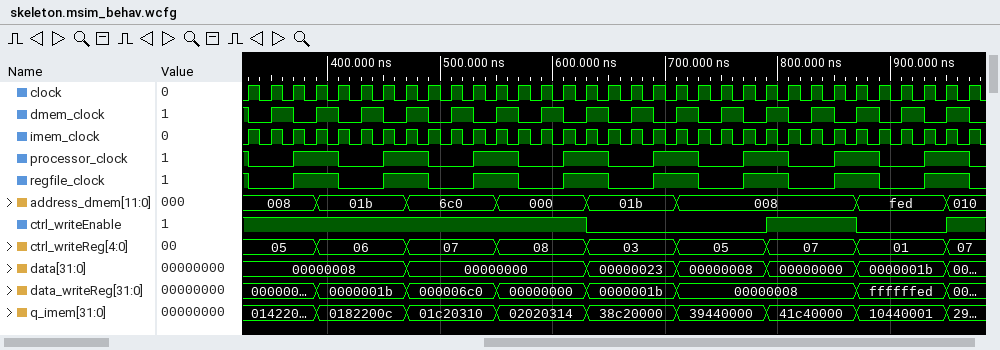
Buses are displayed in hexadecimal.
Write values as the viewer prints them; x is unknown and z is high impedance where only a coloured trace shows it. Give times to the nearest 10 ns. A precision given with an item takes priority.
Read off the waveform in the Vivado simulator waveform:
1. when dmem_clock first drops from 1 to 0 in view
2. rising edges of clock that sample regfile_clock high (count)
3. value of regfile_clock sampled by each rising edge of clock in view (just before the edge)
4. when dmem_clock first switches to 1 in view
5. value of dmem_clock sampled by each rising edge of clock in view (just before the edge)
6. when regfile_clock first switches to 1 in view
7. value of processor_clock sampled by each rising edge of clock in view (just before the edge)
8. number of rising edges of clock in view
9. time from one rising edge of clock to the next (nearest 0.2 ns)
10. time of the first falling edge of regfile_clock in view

330 ns
17
1 0 0 1 1 0 0 1 1 0 0 1 1 0 0 1 1 0 0 1 1 0 0 1 1 0 0 1 1 0 0 1 1
350 ns
1 0 1 0 1 0 1 0 1 0 1 0 1 0 1 0 1 0 1 0 1 0 1 0 1 0 1 0 1 0 1 0 1
370 ns
1 0 0 1 1 0 0 1 1 0 0 1 1 0 0 1 1 0 0 1 1 0 0 1 1 0 0 1 1 0 0 1 1
33
20 ns
330 ns
